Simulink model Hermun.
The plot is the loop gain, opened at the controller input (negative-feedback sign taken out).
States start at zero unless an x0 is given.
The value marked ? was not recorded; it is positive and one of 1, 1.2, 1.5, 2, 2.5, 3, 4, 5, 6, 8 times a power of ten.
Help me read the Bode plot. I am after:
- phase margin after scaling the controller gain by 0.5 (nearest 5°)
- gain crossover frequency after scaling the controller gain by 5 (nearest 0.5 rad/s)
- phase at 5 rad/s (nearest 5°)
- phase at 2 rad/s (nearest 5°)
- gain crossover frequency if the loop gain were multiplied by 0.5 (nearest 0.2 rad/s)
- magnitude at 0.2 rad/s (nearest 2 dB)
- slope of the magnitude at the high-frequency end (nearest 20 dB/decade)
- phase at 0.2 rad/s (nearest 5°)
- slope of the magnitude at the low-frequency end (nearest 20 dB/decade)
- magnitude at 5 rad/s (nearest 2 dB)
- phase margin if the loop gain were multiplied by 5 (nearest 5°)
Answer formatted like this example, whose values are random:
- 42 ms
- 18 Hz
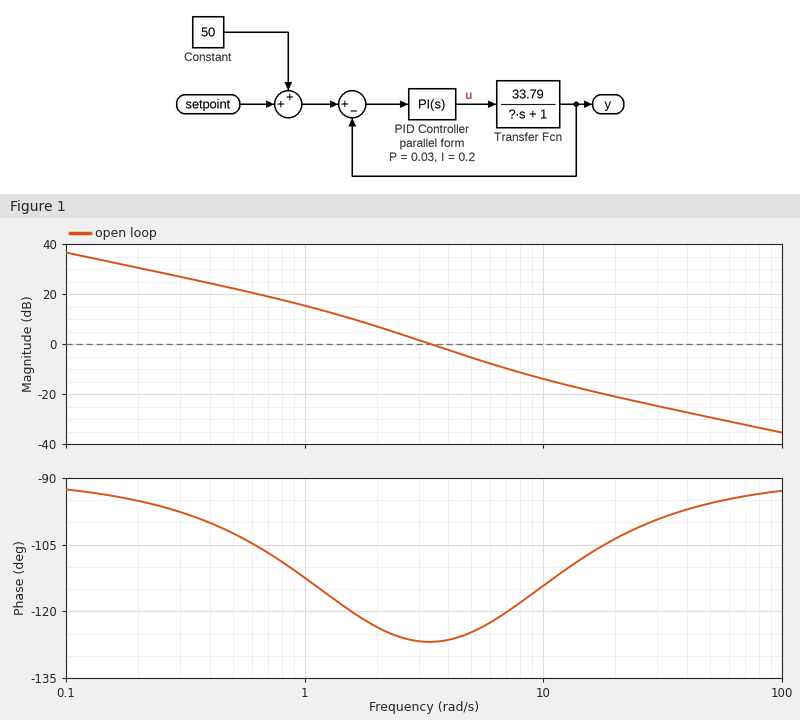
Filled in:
- 55°
- 10.0 rad/s
- -125°
- -125°
- 2.2 rad/s
- 30 dB
- -20 dB/decade
- -95°
- -20 dB/decade
- -6 dB
- 65°
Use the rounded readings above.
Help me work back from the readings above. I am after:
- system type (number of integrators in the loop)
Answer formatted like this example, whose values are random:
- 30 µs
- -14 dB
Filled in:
- 1
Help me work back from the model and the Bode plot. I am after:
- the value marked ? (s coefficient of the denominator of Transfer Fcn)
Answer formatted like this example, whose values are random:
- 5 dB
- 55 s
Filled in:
- 0.6
